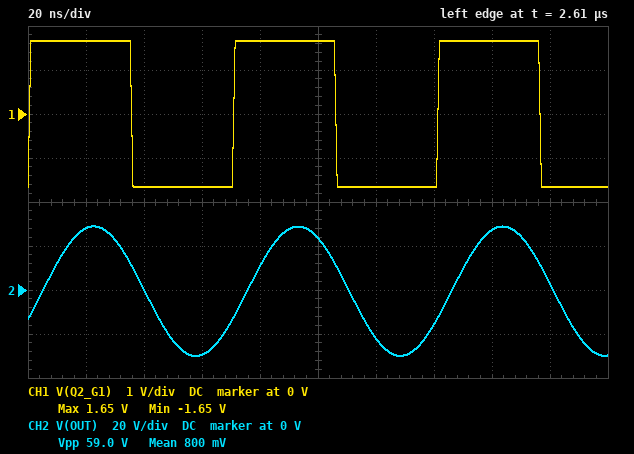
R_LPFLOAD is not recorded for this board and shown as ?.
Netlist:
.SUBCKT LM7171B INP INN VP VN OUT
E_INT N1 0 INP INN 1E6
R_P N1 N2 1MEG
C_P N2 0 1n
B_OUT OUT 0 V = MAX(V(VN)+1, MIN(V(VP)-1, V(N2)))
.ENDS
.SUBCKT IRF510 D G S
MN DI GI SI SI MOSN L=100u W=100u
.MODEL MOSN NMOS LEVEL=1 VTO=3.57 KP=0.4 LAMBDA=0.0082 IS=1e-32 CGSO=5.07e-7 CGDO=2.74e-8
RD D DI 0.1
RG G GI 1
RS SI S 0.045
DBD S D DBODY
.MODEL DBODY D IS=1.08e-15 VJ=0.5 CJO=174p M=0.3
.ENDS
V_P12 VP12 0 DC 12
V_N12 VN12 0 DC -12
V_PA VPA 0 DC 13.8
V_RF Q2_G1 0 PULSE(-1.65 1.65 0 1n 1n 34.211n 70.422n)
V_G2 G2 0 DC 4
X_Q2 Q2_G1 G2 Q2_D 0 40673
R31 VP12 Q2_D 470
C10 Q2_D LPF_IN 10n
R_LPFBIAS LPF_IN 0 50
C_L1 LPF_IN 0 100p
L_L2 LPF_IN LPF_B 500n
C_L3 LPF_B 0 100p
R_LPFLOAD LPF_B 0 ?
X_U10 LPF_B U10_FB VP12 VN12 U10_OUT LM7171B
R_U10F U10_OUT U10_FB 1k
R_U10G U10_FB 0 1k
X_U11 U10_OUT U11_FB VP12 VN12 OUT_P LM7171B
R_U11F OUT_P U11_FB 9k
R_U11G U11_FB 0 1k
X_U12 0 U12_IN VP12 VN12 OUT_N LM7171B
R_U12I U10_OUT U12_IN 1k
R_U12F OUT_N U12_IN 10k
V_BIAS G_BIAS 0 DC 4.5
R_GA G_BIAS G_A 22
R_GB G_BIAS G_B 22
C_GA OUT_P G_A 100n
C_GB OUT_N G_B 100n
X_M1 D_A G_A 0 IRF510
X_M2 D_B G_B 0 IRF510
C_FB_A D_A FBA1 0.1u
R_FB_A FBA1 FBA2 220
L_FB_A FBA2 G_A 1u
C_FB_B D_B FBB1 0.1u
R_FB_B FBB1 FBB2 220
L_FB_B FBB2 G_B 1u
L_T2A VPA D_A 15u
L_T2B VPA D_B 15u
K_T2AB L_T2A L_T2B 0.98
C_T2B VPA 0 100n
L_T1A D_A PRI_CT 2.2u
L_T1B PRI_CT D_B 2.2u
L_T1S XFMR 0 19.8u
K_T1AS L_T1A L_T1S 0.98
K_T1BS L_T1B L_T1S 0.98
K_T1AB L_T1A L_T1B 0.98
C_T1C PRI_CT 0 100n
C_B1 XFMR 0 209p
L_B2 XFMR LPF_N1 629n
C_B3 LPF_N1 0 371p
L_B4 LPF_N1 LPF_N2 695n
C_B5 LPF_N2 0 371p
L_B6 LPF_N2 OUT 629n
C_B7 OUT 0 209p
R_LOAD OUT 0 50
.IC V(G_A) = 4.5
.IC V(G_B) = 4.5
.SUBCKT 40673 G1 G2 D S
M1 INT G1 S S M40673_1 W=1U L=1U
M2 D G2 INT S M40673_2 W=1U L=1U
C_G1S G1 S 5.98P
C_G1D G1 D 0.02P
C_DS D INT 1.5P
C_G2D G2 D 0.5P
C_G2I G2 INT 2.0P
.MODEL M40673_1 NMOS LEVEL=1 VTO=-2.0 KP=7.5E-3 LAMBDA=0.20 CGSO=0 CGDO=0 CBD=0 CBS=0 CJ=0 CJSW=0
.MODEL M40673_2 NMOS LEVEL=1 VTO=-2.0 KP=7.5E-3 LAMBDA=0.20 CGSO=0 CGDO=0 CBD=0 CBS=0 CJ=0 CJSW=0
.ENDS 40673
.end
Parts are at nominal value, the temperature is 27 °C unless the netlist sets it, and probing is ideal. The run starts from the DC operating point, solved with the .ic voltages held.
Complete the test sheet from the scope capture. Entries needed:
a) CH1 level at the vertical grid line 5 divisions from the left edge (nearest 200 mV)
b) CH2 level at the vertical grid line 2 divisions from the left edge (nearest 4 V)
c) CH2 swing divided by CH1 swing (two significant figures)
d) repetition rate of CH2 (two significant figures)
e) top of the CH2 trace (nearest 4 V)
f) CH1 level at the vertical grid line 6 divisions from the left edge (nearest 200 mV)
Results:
1.6 V
0 V
18
14 MHz
28 V
-1.6 V
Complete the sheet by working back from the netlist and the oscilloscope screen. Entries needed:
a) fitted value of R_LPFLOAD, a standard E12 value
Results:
15 Ω
